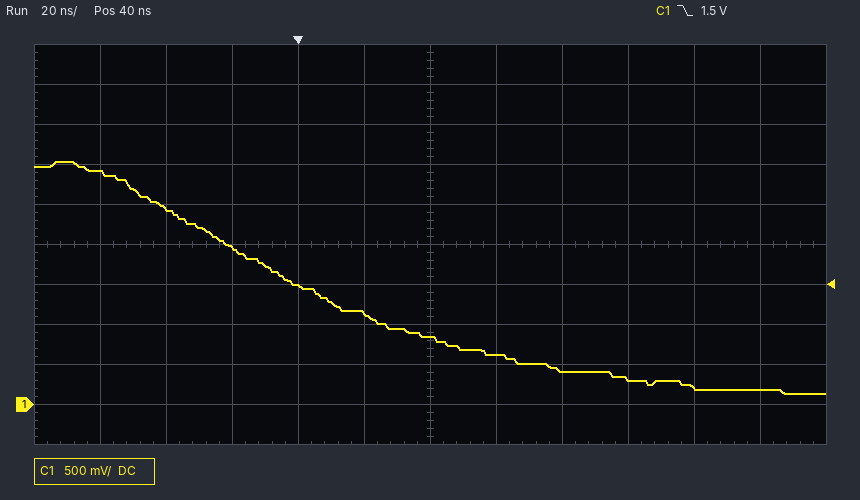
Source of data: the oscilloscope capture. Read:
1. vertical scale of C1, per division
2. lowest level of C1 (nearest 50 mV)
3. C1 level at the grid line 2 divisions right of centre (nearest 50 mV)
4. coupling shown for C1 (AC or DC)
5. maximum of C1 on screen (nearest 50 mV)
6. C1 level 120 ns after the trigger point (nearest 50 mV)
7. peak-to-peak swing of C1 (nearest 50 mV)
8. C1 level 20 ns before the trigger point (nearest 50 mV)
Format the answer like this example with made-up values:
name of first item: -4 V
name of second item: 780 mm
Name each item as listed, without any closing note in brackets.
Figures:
vertical scale of C1, per division: 500 mV
lowest level of C1: 150 mV
C1 level at the grid line 2 divisions right of centre: 400 mV
coupling shown for C1: DC
maximum of C1 on screen: 3.05 V
C1 level 120 ns after the trigger point: 200 mV
peak-to-peak swing of C1: 2.90 V
C1 level 20 ns before the trigger point: 1.95 V
